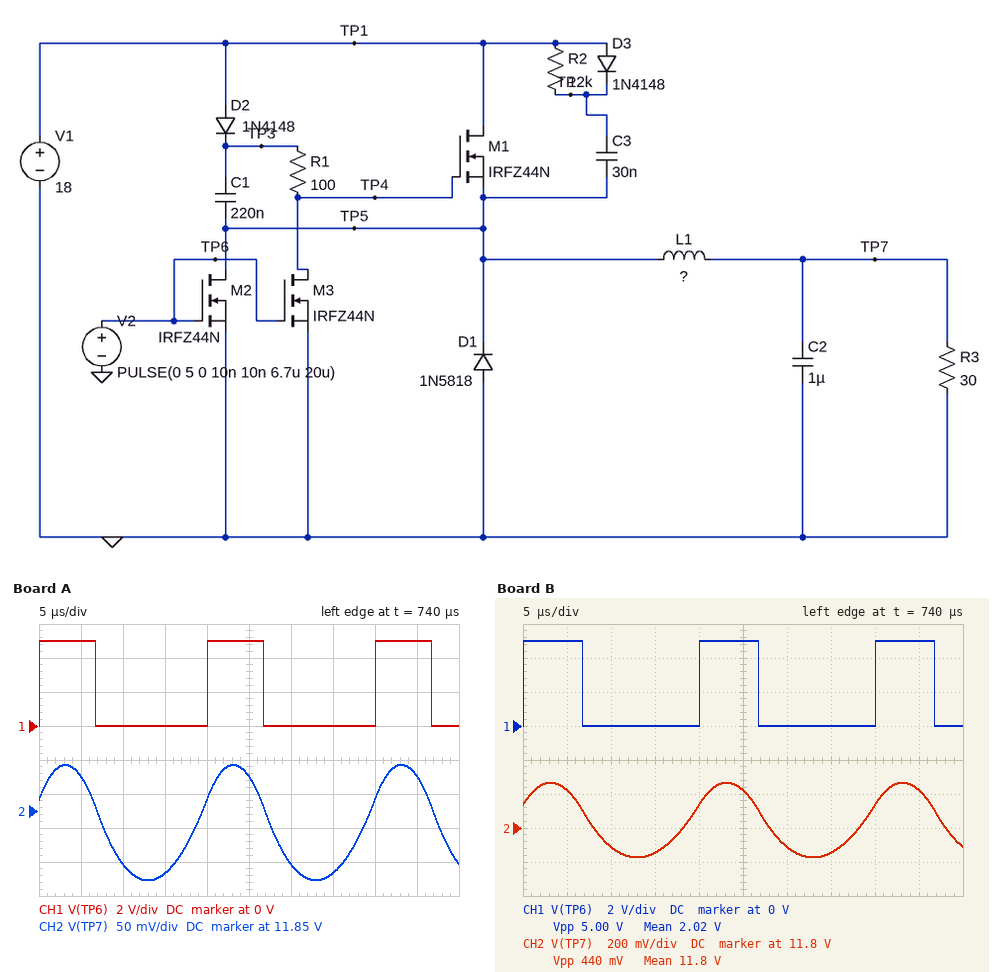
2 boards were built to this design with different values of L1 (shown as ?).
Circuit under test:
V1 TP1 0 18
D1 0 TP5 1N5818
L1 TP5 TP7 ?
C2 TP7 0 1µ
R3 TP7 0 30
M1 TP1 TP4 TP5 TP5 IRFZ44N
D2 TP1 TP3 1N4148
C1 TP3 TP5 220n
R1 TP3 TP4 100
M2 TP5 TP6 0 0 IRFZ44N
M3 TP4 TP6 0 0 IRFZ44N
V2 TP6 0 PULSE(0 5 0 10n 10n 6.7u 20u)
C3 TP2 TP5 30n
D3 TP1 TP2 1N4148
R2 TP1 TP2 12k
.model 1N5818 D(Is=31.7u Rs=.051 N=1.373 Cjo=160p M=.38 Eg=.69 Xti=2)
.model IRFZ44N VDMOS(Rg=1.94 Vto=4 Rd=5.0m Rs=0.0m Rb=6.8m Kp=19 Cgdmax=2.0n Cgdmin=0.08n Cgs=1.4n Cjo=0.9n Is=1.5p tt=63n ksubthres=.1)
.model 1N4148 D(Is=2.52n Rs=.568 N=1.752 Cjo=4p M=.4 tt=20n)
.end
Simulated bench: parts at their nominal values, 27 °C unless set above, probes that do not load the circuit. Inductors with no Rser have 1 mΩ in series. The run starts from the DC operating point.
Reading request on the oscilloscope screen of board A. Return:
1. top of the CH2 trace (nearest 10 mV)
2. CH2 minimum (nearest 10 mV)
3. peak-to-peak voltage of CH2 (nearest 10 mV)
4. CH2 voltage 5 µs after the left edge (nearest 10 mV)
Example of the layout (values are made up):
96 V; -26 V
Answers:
11.92 V; 11.75 V; 170 mV; 11.90 V
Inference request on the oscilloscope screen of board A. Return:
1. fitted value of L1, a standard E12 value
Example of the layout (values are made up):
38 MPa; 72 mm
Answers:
1.2 mH
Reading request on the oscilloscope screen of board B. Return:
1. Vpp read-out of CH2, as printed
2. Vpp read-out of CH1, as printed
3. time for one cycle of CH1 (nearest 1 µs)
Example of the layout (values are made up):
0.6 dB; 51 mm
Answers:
440 mV; 5.00 V; 20 µs
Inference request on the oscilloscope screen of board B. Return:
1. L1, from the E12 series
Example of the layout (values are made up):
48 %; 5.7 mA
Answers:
470 µH
